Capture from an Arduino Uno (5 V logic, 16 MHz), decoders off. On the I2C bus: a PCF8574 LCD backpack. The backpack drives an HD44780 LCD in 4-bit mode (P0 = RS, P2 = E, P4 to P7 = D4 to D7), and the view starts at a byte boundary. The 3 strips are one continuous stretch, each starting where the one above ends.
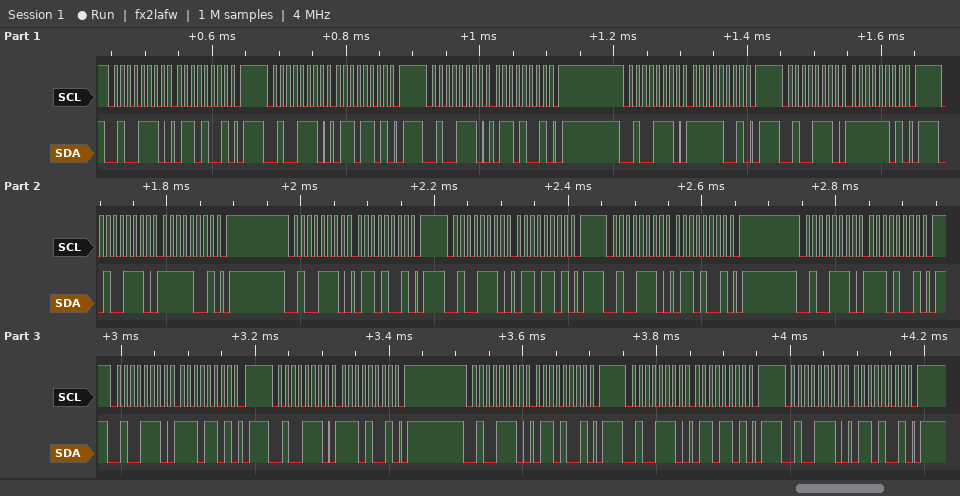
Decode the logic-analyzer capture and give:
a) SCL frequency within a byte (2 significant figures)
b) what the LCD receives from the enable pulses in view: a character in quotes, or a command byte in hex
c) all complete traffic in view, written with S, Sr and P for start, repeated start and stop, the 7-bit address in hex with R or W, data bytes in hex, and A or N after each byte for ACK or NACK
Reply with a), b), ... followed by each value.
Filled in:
a) 100 kHz
b) 'o' 'n'
c) S 27W A 69 A P S 27W A 6D A P S 27W A 69 A P S 27W A F9 A P S 27W A FD A P S 27W A F9 A P S 27W A 69 A P S 27W A 6D A P S 27W A 69 A P S 27W A E9 A P S 27W A ED A P S 27W A E9 A P S 27W A 69 A P S 27W A 6D A P S 27W A 69 A P
